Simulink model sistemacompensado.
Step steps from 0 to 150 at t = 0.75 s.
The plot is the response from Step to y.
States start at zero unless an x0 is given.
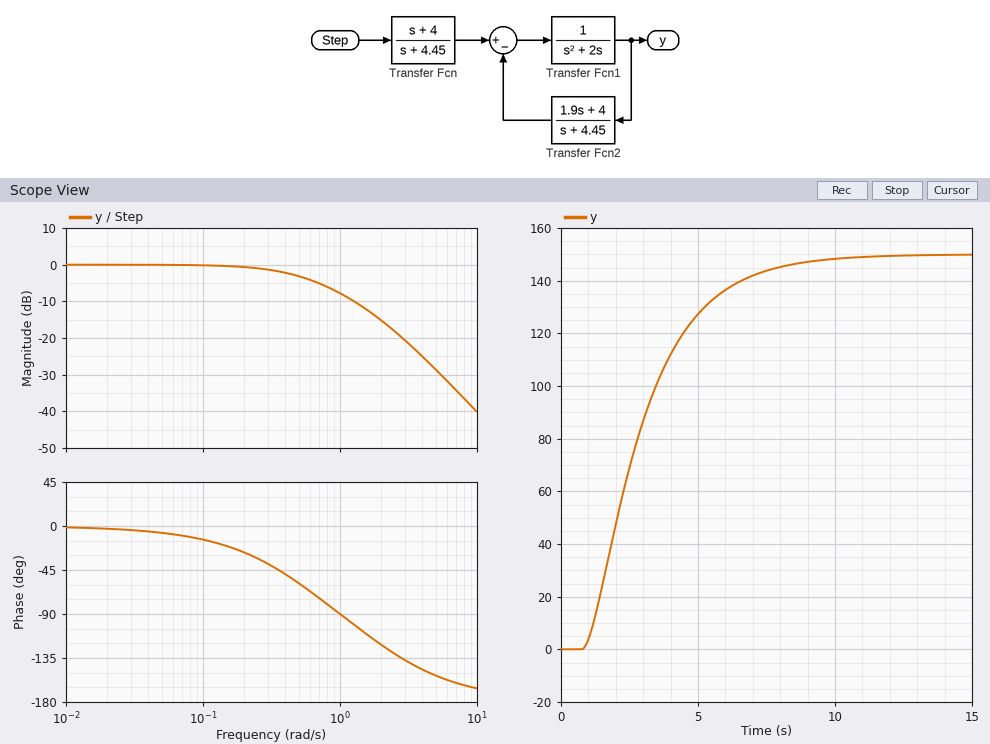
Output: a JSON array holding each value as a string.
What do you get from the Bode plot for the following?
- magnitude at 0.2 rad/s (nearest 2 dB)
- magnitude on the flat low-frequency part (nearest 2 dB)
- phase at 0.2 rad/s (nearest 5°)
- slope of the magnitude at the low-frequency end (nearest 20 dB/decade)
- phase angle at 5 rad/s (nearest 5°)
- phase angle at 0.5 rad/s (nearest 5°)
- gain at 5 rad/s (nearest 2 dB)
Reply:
["0 dB", "0 dB", "-25°", "0 dB/decade", "-155°", "-60°", "-28 dB"]
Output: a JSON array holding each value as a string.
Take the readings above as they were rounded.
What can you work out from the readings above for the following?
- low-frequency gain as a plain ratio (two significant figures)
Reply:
["1.0"]
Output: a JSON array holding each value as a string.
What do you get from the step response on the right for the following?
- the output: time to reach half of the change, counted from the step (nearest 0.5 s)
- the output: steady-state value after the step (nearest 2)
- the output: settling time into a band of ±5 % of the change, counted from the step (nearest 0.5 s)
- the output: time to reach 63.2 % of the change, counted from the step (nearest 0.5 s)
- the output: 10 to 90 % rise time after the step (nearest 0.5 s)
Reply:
["2.0 s", "150", "6.5 s", "2.5 s", "4.5 s"]
